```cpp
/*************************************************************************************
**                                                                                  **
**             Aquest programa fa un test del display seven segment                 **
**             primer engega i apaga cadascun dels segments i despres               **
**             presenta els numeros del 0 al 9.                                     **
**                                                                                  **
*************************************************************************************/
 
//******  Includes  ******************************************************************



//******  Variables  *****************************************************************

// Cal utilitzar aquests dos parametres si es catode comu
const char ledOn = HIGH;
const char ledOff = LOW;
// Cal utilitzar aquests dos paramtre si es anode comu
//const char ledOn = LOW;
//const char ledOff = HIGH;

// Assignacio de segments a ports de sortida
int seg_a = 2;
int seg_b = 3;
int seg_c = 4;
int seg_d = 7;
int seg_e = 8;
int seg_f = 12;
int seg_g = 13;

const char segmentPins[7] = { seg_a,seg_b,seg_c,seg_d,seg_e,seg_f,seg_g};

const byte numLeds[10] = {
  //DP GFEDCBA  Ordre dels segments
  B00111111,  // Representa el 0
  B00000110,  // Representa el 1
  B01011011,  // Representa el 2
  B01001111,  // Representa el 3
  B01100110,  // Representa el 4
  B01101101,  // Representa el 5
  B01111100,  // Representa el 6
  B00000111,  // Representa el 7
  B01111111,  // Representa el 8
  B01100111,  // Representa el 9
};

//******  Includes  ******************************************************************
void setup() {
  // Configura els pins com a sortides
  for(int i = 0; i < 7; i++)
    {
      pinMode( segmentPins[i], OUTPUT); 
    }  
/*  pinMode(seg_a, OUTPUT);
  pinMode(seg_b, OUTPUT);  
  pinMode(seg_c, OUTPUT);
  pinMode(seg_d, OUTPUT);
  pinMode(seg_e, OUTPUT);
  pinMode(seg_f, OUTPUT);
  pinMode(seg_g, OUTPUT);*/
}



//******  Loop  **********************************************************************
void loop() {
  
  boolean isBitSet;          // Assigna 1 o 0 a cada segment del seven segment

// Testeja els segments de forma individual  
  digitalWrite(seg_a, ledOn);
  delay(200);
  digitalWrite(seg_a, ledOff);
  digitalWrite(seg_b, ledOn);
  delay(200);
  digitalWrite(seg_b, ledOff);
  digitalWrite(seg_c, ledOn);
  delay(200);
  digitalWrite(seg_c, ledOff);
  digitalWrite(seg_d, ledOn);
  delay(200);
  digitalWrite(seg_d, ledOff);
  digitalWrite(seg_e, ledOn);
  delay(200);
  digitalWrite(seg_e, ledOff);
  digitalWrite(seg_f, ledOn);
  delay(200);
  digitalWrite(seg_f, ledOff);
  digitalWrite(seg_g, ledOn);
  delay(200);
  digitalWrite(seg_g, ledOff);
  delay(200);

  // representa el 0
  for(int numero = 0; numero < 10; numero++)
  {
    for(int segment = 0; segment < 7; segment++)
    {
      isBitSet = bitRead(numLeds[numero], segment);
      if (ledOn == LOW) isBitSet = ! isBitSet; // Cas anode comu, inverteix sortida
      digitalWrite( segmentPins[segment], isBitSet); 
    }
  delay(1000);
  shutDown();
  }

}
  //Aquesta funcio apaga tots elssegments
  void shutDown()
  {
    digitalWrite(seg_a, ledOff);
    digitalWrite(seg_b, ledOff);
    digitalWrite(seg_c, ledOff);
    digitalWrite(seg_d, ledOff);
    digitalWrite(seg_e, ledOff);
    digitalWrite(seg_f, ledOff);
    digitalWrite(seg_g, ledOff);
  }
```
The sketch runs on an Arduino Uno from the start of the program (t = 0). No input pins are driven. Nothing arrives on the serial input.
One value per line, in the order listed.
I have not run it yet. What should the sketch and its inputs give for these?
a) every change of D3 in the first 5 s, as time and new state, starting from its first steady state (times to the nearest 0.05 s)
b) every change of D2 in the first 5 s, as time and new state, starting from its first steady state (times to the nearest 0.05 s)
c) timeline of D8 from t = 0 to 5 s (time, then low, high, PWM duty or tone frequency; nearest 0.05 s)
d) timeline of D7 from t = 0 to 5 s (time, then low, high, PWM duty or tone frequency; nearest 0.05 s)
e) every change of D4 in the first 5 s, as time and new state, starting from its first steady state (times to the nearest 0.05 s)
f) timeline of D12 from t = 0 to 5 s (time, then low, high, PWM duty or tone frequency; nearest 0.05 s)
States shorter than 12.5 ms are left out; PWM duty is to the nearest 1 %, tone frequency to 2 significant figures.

0 s low; 0.2 s high; 0.4 s low; 1.6 s high
0 s high; 0.2 s low; 1.6 s high; 2.6 s low; 3.6 s high
0 s low; 0.8 s high; 1 s low; 1.6 s high; 2.6 s low; 3.6 s high; 4.6 s low
0 s low; 0.6 s high; 0.8 s low; 1.6 s high; 2.6 s low; 3.6 s high
0 s low; 0.4 s high; 0.6 s low; 1.6 s high; 3.6 s low; 4.6 s high
0 s low; 1 s high; 1.2 s low; 1.6 s high; 2.6 s low
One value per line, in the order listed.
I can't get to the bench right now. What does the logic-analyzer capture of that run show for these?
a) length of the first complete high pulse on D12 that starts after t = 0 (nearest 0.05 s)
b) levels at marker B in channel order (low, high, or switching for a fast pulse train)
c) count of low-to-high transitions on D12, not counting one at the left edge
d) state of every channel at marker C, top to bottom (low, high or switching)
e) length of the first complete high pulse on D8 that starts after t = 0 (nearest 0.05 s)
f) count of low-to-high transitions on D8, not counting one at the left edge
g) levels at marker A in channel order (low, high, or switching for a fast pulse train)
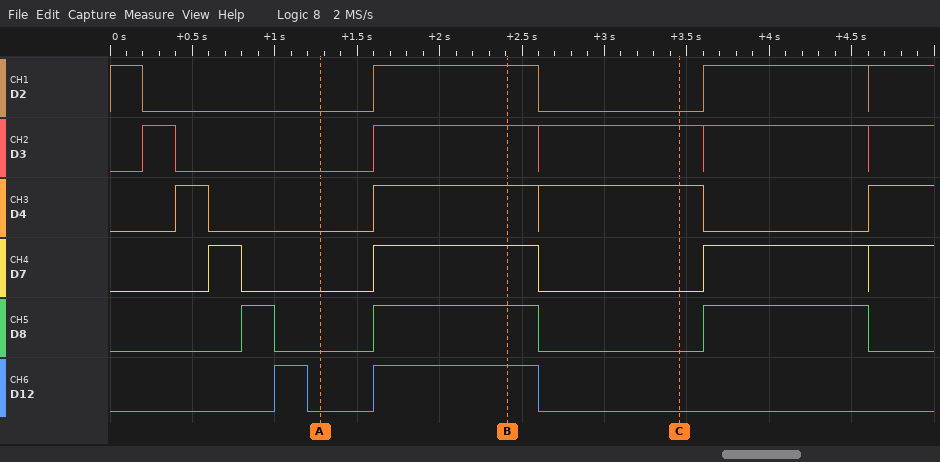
0.20 s
D2 high, D3 high, D4 high, D7 high, D8 high, D12 high
2
D2 low, D3 high, D4 high, D7 low, D8 low, D12 low
0.20 s
3
D2 low, D3 low, D4 low, D7 low, D8 low, D12 low
